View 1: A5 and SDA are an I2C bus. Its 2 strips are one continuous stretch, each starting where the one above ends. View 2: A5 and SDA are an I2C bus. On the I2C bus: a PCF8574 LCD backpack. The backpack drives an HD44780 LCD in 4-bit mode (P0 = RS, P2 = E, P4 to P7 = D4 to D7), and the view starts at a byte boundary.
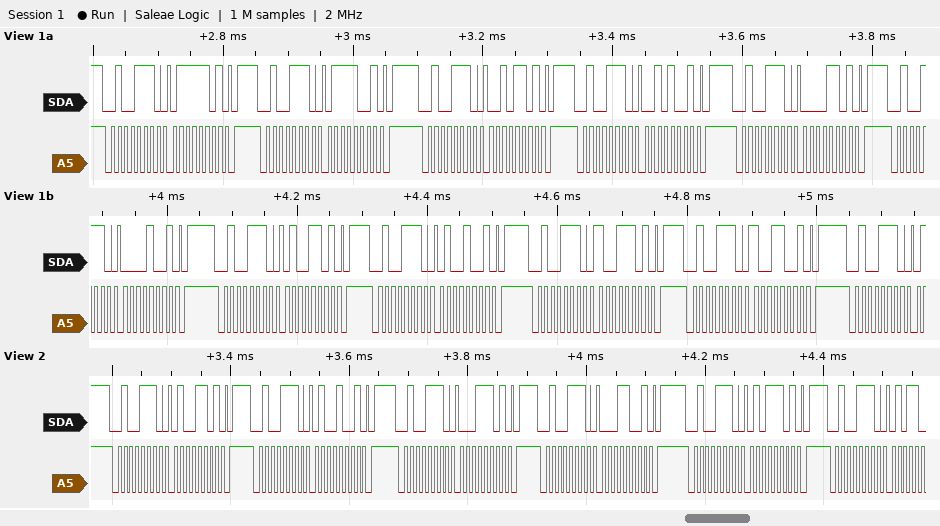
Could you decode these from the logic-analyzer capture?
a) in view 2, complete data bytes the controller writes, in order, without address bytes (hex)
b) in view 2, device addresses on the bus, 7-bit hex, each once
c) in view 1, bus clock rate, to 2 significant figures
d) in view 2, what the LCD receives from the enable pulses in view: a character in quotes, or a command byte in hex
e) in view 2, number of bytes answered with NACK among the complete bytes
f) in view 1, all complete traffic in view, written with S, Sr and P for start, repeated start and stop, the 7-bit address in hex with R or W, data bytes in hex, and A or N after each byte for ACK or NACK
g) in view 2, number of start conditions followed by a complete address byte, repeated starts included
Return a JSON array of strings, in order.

["4D 49 1D 19 5D", "0x27", "100 kHz", "'A'", "0", "S 27W A 7D A P S 27W A 79 A P S 27W A 2D A P S 27W A 29 A P S 27W A 0D A P S 27W A 09 A P S 27W A 4D A P S 27W A 49 A P S 27W A 9D A P S 27W A 99 A P S 27W A", "6"]
